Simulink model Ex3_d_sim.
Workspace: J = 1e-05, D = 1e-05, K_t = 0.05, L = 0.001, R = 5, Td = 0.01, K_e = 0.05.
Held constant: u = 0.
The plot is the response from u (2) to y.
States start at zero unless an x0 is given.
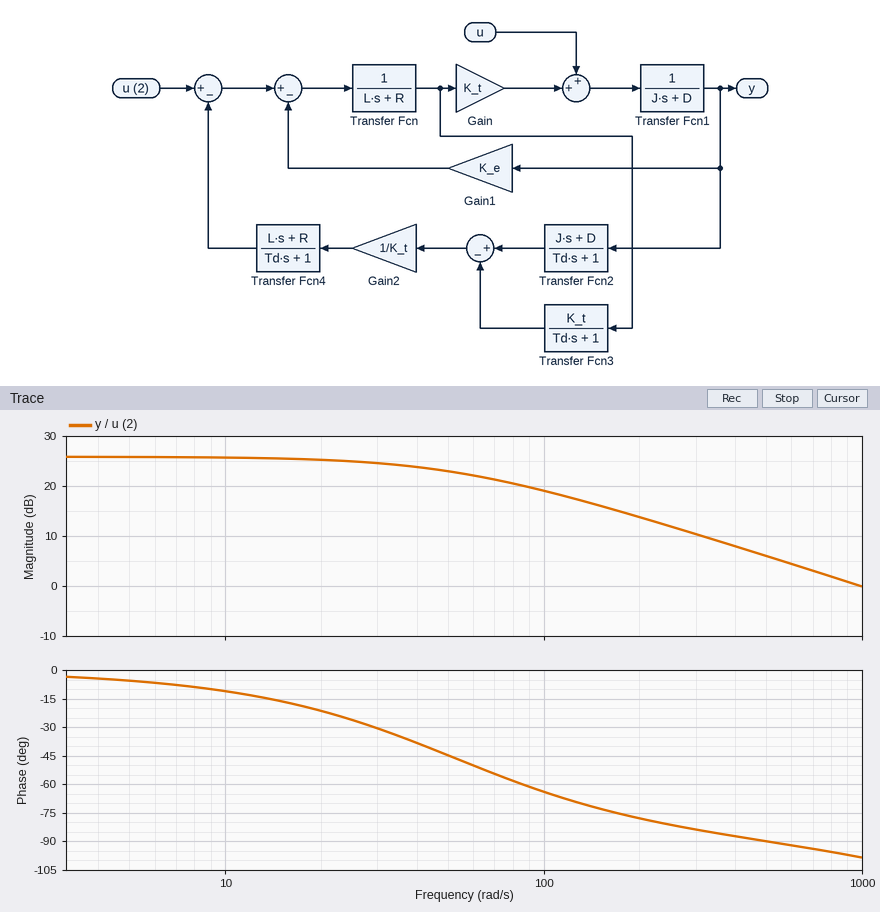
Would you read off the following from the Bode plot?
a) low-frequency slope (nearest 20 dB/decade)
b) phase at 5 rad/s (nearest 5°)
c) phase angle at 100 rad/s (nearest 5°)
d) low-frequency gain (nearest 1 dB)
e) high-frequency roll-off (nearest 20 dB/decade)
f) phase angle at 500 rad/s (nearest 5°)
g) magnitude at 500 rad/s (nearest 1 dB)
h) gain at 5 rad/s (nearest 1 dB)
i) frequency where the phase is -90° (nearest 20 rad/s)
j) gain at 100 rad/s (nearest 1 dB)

0 dB/decade
-5°
-65°
26 dB
-20 dB/decade
-90°
6 dB
26 dB
500 rad/s
19 dB
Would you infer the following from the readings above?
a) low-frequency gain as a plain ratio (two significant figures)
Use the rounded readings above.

20
